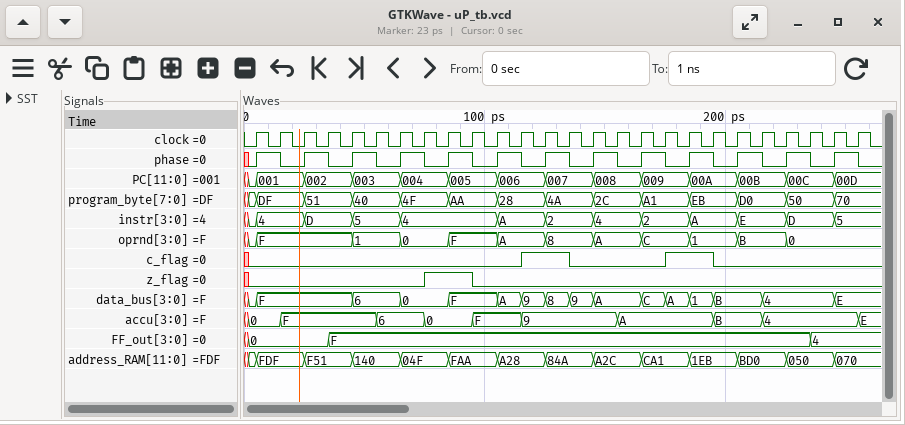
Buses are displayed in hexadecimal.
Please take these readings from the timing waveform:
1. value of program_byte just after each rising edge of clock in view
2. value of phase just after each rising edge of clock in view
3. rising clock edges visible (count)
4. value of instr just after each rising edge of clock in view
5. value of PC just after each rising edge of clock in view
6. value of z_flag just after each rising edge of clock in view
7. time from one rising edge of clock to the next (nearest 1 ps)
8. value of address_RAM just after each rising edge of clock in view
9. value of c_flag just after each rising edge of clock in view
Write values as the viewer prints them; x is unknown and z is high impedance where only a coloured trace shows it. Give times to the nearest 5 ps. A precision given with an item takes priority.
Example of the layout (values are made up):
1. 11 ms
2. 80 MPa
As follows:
1. DF, DF, 51, 51, 40, 40, 4F, 4F, AA, AA, 28, 28, 4A, 4A, 2C, 2C, A1, A1, EB, EB, D0, D0, 50, 50, 70, 70
2. 1 0 1 0 1 0 1 0 1 0 1 0 1 0 1 0 1 0 1 0 1 0 1 0 1 0
3. 26
4. 4, 4, D, D, 5, 5, 4, 4, 4, 4, A, A, 2, 2, 4, 4, 2, 2, A, A, E, E, D, D, 5, 5
5. 001, 001, 002, 002, 003, 003, 004, 004, 005, 005, 006, 006, 007, 007, 008, 008, 009, 009, 00A, 00A, 00B, 00B, 00C, 00C, 00D, 00D
6. 0 0 0 0 0 0 0 1 1 0 0 0 0 0 0 0 0 0 0 0 0 0 0 0 0 0
7. 10 ps
8. FDF, FDF, F51, F51, 140, 140, 04F, 04F, FAA, FAA, A28, A28, 84A, 84A, A2C, A2C, CA1, CA1, 1EB, 1EB, BD0, BD0, 050, 050, 070, 070
9. 0 0 0 0 0 0 0 0 0 0 0 1 1 0 0 0 0 1 1 0 0 0 0 0 0 0
